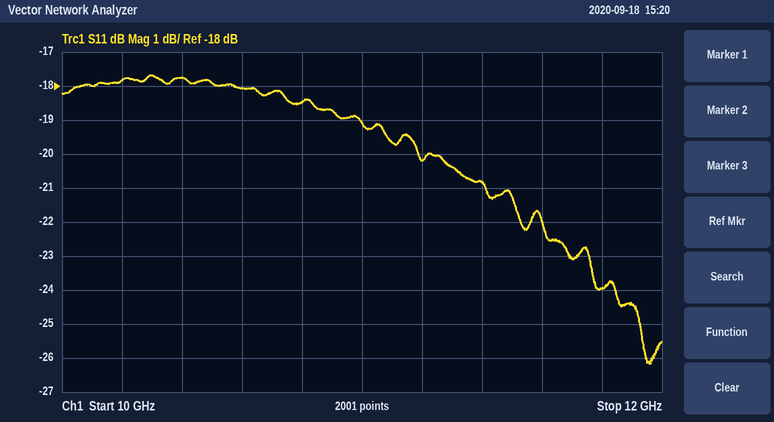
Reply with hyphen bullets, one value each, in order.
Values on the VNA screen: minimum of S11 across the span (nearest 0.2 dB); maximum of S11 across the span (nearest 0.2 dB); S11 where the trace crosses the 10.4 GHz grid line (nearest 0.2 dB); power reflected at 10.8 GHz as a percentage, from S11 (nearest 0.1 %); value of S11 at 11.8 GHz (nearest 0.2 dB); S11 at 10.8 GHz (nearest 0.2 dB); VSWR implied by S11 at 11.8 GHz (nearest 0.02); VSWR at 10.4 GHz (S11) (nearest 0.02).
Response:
- -26.2 dB
- -17.6 dB
- -17.8 dB
- 1.4 %
- -24.0 dB
- -18.4 dB
- 1.14
- 1.30
